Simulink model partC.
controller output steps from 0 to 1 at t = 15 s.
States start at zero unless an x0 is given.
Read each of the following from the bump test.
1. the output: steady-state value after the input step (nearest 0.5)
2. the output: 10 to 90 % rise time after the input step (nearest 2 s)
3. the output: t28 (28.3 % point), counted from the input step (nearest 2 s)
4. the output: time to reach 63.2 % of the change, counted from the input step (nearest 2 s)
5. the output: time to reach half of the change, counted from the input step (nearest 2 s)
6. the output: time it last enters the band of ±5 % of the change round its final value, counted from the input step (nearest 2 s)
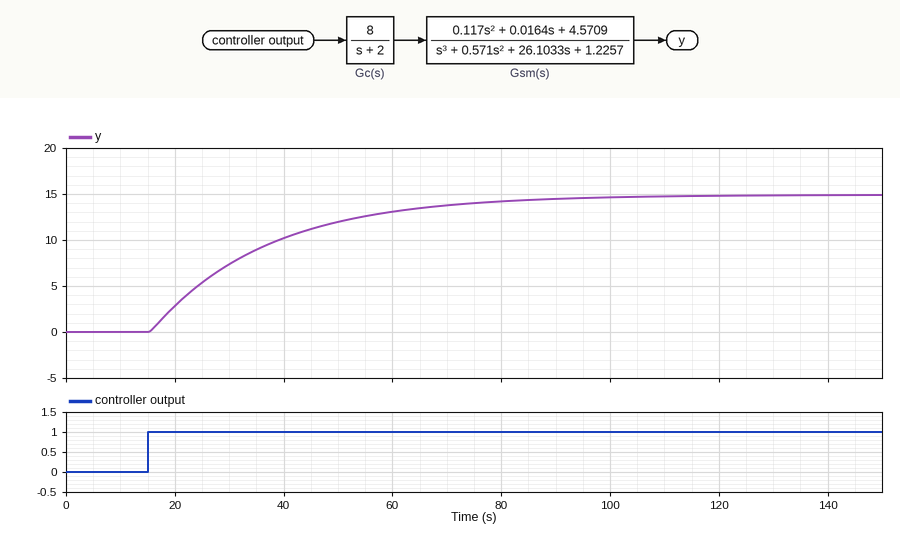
15.0
46 s
8 s
22 s
16 s
64 s
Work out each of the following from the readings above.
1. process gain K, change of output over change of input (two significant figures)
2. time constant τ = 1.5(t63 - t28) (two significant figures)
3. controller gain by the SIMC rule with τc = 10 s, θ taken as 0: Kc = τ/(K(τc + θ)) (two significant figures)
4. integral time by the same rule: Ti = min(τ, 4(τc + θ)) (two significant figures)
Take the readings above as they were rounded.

15
21 s
0.14
21 s
